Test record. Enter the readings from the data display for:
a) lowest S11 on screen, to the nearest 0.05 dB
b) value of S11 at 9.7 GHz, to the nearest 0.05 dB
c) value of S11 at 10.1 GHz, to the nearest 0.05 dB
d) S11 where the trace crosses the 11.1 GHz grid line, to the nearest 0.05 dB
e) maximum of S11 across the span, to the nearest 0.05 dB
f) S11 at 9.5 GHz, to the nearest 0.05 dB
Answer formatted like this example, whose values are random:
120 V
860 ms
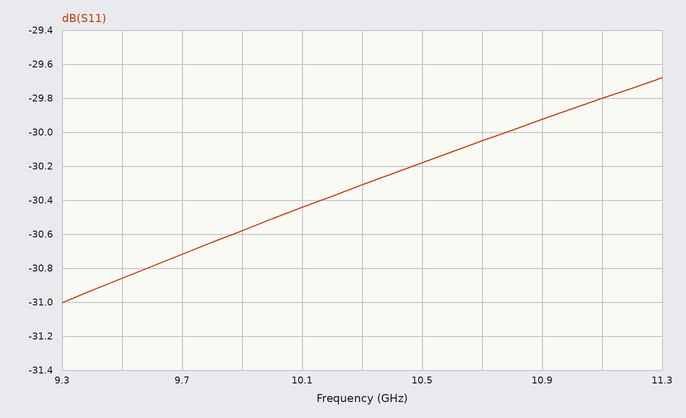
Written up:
-31.00 dB
-30.70 dB
-30.45 dB
-29.80 dB
-29.70 dB
-30.85 dB
